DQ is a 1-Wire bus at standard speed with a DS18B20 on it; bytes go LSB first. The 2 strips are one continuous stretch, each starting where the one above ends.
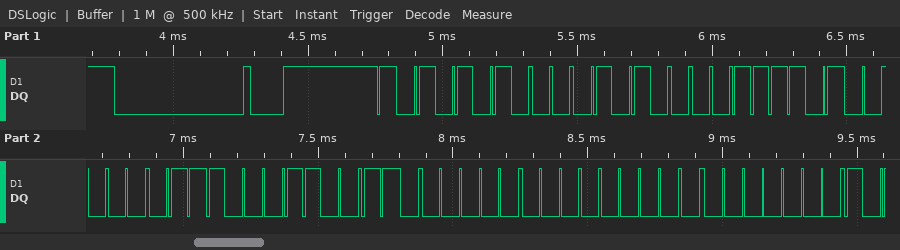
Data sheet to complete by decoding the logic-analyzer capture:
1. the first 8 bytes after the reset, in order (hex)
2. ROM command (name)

55 28 BC C0 31 03 00 00
Match ROM
